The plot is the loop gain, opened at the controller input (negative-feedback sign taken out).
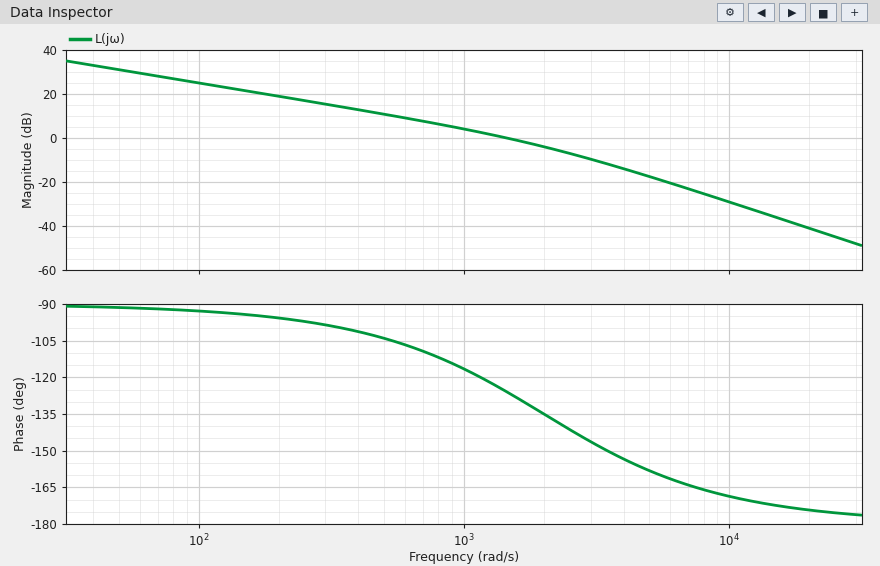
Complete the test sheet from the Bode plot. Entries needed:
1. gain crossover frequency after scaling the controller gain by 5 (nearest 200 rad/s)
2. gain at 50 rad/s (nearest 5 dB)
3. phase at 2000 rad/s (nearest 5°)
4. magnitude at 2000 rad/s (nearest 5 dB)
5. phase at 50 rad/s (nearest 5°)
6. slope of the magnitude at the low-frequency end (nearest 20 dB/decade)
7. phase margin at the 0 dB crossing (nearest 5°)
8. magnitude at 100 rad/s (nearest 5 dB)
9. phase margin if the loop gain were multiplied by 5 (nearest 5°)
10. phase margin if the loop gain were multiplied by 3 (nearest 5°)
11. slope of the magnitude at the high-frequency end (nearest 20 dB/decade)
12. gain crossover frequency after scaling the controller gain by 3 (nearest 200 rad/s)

4000 rad/s
30 dB
-135°
-5 dB
-90°
-20 dB/decade
55°
25 dB
25°
35°
-40 dB/decade
3000 rad/s
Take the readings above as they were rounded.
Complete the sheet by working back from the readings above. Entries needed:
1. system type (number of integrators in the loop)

1
